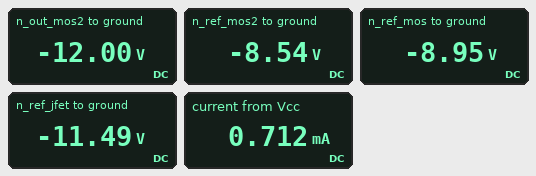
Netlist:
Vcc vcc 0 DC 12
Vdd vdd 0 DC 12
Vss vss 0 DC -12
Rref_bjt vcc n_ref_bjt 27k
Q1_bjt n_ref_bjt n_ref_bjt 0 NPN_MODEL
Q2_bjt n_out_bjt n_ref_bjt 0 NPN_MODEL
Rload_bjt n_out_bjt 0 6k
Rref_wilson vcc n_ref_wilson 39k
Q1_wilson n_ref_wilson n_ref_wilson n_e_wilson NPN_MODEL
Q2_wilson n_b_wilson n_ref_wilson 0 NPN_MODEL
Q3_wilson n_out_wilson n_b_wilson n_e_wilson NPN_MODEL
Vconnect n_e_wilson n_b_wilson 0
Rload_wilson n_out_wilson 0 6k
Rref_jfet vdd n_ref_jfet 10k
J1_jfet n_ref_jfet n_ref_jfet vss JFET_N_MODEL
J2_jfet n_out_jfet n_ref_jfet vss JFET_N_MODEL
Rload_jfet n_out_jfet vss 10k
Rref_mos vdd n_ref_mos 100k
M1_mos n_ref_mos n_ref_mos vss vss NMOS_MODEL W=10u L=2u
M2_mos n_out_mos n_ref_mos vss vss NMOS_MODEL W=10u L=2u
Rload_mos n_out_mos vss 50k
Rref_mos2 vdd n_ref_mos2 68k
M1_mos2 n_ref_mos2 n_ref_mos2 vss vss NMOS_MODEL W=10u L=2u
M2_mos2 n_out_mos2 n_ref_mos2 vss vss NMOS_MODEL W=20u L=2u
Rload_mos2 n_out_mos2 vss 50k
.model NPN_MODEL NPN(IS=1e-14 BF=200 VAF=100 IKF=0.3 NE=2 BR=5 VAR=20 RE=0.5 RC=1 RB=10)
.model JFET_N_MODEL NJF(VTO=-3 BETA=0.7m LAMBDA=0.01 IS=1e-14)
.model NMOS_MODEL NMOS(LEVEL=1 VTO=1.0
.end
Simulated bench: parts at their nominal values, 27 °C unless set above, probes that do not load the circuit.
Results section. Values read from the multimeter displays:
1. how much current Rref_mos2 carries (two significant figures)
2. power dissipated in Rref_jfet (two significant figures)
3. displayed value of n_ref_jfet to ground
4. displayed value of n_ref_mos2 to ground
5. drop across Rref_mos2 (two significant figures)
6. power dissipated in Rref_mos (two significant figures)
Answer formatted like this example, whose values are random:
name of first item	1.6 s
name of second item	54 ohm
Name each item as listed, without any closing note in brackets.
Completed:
how much current Rref_mos2 carries	300 µA
power dissipated in Rref_jfet	55 mW
displayed value of n_ref_jfet to ground	-11.49 V
displayed value of n_ref_mos2 to ground	-8.54 V
drop across Rref_mos2	21 V
power dissipated in Rref_mos	4.4 mW
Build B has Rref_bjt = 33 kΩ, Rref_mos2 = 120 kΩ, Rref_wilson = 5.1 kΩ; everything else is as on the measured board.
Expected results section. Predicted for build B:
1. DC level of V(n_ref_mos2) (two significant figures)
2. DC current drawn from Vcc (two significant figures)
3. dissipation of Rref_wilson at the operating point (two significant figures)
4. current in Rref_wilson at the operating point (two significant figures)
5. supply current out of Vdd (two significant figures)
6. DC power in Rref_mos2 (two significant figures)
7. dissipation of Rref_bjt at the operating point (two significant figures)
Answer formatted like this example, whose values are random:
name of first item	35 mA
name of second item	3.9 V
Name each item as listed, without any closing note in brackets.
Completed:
DC level of V(n_ref_mos2)	-9.1 V
DC current drawn from Vcc	2.6 mA
dissipation of Rref_wilson at the operating point	25 mW
current in Rref_wilson at the operating point	2.2 mA
supply current out of Vdd	2.7 mA
DC power in Rref_mos2	3.7 mW
dissipation of Rref_bjt at the operating point	3.9 mW
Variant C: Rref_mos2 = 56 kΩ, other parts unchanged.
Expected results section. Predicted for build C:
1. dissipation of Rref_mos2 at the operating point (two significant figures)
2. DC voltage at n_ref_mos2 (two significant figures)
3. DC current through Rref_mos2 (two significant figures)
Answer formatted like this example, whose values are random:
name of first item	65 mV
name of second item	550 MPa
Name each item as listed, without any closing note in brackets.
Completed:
dissipation of Rref_mos2 at the operating point	7.4 mW
DC voltage at n_ref_mos2	-8.3 V
DC current through Rref_mos2	360 µA
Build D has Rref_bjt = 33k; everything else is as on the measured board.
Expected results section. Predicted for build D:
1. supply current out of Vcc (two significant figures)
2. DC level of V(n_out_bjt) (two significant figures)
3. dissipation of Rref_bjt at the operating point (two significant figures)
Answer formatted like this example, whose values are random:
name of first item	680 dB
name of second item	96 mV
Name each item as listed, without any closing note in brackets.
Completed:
supply current out of Vcc	640 µA
DC level of V(n_out_bjt)	4.8 mV
dissipation of Rref_bjt at the operating point	3.9 mW
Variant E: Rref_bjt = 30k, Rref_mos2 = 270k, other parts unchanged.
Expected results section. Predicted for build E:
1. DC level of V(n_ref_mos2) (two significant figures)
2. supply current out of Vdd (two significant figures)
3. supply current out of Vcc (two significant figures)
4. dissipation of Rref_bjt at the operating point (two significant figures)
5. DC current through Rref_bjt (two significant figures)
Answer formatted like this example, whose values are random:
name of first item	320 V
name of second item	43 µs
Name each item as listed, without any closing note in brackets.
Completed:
DC level of V(n_ref_mos2)	-9.7 V
supply current out of Vdd	2.6 mA
supply current out of Vcc	670 µA
dissipation of Rref_bjt at the operating point	4.3 mW
DC current through Rref_bjt	380 µA
